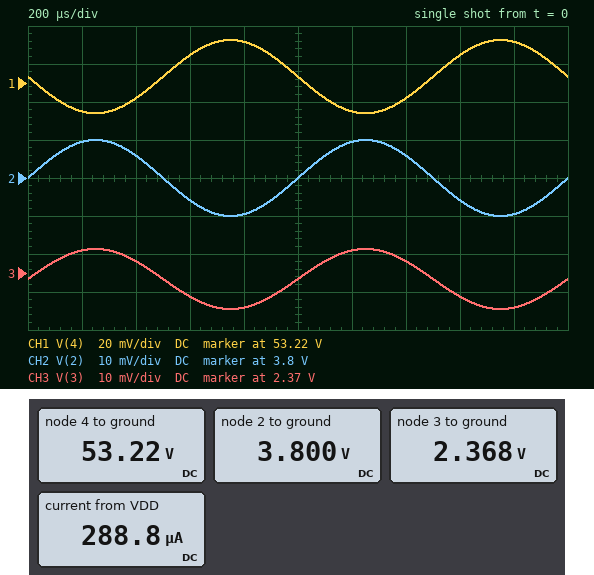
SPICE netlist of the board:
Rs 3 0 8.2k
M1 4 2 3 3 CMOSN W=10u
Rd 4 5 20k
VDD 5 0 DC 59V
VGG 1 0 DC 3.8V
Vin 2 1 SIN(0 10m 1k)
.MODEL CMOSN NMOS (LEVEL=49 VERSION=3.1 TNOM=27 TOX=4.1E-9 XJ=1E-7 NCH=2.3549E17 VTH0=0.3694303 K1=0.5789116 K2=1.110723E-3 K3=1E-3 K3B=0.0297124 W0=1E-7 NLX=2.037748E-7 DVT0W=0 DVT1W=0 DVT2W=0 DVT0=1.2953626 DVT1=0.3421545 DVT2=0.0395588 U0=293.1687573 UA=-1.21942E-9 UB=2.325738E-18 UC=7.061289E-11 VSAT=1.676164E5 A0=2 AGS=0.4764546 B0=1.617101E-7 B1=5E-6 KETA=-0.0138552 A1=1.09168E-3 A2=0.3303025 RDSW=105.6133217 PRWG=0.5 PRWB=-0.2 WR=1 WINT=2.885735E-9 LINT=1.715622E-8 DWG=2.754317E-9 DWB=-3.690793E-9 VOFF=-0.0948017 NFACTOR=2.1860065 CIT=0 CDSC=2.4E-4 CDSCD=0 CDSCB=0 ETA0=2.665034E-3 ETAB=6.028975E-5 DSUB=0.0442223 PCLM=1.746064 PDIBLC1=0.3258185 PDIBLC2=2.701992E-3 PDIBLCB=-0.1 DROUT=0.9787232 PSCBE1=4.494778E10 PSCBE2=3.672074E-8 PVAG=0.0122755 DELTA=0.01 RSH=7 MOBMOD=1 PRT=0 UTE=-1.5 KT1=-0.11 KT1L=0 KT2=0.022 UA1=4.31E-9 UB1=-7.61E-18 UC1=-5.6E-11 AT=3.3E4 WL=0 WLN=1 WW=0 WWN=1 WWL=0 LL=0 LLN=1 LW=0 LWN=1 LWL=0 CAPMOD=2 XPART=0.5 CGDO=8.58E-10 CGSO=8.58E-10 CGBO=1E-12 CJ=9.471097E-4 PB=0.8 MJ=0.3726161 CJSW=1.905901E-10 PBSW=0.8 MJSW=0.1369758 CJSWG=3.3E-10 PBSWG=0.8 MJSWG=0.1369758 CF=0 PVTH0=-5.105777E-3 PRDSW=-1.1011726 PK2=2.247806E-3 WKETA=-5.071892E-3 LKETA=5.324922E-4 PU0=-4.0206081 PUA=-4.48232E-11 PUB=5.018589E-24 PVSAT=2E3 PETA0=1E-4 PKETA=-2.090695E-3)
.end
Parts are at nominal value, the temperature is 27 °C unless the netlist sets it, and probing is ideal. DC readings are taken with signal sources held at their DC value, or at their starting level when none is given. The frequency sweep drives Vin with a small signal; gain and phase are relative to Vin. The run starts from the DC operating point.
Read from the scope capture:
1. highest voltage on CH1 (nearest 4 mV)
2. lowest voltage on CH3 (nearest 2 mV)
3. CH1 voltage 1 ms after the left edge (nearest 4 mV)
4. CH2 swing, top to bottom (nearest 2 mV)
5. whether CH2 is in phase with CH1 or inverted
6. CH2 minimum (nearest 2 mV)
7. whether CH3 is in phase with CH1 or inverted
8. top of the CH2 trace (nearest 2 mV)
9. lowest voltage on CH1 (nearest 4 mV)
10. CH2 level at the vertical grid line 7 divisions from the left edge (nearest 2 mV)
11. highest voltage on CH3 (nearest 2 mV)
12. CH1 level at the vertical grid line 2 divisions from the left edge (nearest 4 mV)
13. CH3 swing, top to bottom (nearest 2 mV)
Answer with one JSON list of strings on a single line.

["53.244 V", "2.360 V", "53.224 V", "20 mV", "inverted", "3.790 V", "inverted", "3.810 V", "53.204 V", "3.806 V", "2.376 V", "53.212 V", "16 mV"]
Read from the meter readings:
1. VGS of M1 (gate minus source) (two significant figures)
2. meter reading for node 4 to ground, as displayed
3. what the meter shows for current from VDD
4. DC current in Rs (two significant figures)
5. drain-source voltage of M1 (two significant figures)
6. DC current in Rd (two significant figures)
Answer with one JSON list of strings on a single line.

["1.4 V", "53.22 V", "288.8 µA", "290 µA", "51 V", "290 µA"]
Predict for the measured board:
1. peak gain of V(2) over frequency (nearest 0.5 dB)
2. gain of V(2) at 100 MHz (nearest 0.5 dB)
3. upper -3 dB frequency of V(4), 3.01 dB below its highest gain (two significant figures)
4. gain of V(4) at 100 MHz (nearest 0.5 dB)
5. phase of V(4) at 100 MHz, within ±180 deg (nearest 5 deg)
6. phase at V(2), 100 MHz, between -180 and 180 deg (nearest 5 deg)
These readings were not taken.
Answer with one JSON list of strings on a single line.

["0 dB", "0 dB", "1.3 GHz", "6.0 dB", "145 deg", "0 deg"]
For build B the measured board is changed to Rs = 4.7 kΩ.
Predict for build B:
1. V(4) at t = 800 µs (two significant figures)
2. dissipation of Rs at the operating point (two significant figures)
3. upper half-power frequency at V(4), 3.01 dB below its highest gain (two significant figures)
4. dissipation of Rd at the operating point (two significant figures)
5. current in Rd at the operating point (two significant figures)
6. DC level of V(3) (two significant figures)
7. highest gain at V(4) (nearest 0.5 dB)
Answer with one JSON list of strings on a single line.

["50 V", "910 µW", "1.2 GHz", "3.9 mW", "440 µA", "2.1 V", "10.0 dB"]
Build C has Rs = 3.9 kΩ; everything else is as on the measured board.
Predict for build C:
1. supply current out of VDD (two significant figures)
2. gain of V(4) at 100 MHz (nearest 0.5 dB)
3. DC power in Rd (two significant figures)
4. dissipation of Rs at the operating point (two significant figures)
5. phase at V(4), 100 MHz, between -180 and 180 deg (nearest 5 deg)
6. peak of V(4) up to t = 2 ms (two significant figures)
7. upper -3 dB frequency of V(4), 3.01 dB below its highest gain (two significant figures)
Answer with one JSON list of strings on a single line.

["500 µA", "11.0 dB", "5.0 mW", "980 µW", "155 deg", "49 V", "1.2 GHz"]
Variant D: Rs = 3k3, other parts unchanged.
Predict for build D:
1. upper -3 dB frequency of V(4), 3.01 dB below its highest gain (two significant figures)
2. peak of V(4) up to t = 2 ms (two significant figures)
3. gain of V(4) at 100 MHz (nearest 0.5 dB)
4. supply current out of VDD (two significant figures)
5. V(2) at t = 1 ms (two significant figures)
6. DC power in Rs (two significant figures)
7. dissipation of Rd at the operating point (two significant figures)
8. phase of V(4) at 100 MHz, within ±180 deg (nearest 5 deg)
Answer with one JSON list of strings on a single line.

["1.2 GHz", "48 V", "12.0 dB", "560 µA", "3.8 V", "1.0 mW", "6.3 mW", "155 deg"]
